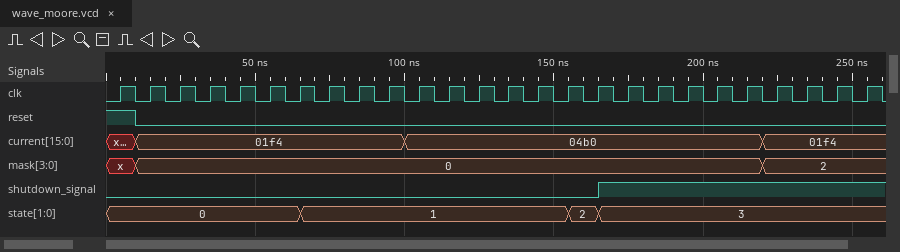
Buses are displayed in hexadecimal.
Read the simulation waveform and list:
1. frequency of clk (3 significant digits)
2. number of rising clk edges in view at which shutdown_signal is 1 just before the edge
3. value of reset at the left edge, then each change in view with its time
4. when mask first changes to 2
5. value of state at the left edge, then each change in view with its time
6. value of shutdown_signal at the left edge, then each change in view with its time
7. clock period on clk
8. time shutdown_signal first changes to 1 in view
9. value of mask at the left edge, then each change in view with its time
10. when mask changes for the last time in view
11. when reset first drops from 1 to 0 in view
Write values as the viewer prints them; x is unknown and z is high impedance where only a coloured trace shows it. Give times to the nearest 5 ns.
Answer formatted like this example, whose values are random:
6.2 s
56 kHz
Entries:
100 MHz
9
1, 0 at 10 ns
220 ns
0, 1 at 65 ns, 2 at 155 ns, 3 at 165 ns
0, 1 at 165 ns
10 ns
165 ns
x, 0 at 10 ns, 2 at 220 ns
220 ns
10 ns
